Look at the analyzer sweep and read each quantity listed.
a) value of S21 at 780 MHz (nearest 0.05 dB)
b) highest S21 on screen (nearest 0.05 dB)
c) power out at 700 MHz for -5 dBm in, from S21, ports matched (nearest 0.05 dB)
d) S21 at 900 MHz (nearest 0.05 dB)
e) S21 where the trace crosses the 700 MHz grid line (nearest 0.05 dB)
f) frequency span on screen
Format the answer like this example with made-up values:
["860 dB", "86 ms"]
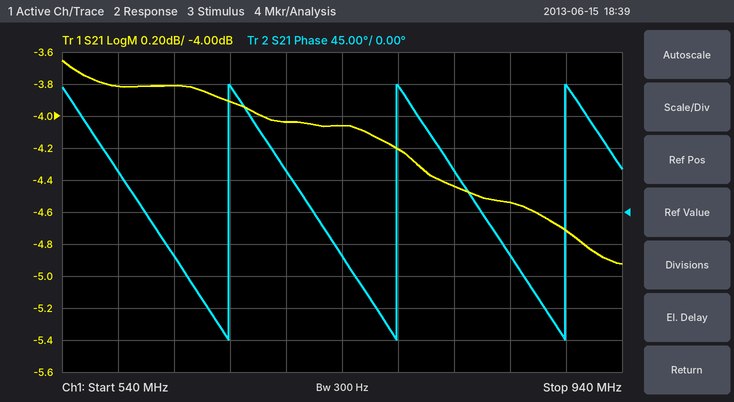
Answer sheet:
["-4.20 dB", "-3.65 dB", "-9.05 dBm", "-4.70 dB", "-4.05 dB", "400 MHz"]
